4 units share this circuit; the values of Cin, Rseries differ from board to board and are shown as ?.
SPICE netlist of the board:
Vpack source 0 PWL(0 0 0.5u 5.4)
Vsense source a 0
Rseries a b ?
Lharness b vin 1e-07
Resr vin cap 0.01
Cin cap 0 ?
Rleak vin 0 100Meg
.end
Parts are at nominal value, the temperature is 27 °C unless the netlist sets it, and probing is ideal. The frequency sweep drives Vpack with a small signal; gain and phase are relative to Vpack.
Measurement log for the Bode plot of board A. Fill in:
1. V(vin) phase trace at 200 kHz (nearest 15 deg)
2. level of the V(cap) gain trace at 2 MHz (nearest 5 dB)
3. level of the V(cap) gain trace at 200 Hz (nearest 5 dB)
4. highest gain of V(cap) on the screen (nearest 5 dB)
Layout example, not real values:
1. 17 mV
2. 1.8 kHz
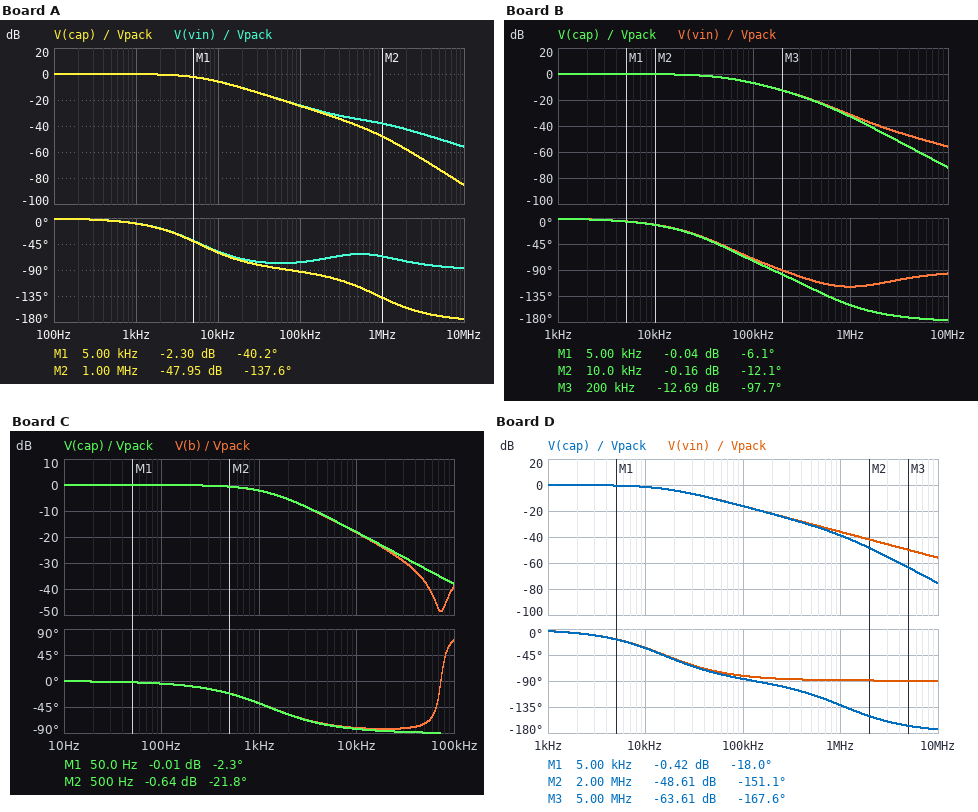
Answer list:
1. -75 deg
2. -60 dB
3. 0 dB
4. 0 dB
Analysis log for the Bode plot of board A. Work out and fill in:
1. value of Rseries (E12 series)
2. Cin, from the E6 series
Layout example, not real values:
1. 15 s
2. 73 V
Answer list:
1. 0.56 Ω
2. 47 µF
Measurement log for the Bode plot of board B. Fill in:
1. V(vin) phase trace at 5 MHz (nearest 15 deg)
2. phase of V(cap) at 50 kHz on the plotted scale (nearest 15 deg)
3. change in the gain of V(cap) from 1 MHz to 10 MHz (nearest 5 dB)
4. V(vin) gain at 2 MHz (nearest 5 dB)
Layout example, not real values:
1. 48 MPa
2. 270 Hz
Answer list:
1. -105 deg
2. -45 deg
3. -40 dB
4. -40 dB
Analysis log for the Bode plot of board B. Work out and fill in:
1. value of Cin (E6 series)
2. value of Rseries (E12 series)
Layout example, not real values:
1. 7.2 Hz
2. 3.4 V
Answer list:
1. 10 µF
2. 0.33 Ω
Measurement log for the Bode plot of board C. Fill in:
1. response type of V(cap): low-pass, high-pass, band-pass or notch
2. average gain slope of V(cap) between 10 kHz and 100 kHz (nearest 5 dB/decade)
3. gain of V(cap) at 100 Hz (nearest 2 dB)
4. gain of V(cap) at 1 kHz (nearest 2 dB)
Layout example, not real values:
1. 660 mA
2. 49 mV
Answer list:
1. low-pass
2. -20 dB/decade
3. 0 dB
4. -2 dB
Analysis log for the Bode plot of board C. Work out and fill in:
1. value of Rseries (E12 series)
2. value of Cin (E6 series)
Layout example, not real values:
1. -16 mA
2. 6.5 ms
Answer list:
1. 2.7 Ω
2. 47 µF
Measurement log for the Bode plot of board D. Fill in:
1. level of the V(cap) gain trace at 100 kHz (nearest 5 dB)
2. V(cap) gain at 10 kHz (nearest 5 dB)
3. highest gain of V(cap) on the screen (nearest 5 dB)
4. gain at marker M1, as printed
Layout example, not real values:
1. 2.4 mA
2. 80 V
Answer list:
1. -15 dB
2. 0 dB
3. 0 dB
4. -0.42 dB
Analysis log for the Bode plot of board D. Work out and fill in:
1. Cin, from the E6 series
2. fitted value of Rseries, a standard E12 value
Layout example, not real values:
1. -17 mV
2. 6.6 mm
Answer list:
1. 15 µF
2. 0.68 Ω
